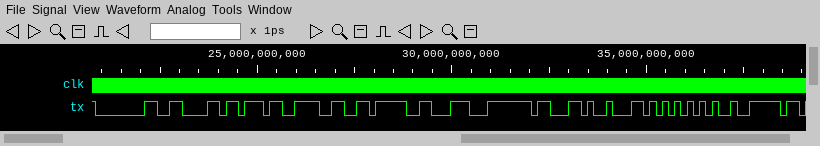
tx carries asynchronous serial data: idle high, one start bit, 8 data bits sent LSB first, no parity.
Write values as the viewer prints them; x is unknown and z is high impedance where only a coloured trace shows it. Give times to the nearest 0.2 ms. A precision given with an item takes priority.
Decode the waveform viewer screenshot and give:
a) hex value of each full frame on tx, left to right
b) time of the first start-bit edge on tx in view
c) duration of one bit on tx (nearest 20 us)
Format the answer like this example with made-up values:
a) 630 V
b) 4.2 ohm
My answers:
a) 80, 86, BB, 9E, F6, C6, FC, 63, 62, 55, F2
b) 20.8 ms
c) 160 us
